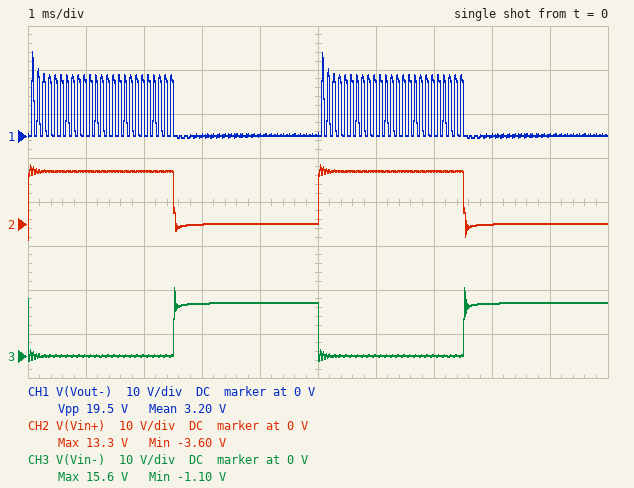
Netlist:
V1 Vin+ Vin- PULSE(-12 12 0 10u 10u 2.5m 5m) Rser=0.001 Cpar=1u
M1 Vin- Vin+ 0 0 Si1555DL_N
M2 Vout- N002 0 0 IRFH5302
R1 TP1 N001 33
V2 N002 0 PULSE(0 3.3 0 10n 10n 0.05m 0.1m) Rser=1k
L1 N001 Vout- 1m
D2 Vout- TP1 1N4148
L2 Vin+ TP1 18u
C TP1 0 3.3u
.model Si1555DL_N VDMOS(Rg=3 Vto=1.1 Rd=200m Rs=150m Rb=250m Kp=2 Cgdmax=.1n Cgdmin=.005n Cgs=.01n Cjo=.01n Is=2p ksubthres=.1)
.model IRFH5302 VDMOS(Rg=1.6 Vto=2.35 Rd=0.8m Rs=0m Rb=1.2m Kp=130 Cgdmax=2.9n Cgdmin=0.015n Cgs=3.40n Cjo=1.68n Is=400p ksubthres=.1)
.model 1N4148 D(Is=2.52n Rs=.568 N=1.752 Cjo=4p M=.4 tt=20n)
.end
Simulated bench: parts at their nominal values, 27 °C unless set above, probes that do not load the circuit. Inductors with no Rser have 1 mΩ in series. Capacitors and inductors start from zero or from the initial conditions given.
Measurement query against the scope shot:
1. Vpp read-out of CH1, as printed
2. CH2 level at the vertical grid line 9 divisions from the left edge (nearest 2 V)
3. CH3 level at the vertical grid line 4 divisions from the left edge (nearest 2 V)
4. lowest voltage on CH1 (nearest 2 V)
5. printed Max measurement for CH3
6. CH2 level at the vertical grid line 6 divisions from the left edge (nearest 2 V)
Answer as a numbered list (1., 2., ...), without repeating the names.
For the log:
1. 19.5 V
2. 0 V
3. 12 V
4. 0 V
5. 15.6 V
6. 12 V
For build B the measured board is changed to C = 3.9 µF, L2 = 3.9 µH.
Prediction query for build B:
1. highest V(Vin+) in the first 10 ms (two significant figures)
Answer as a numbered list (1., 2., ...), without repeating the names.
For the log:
1. 14 V
